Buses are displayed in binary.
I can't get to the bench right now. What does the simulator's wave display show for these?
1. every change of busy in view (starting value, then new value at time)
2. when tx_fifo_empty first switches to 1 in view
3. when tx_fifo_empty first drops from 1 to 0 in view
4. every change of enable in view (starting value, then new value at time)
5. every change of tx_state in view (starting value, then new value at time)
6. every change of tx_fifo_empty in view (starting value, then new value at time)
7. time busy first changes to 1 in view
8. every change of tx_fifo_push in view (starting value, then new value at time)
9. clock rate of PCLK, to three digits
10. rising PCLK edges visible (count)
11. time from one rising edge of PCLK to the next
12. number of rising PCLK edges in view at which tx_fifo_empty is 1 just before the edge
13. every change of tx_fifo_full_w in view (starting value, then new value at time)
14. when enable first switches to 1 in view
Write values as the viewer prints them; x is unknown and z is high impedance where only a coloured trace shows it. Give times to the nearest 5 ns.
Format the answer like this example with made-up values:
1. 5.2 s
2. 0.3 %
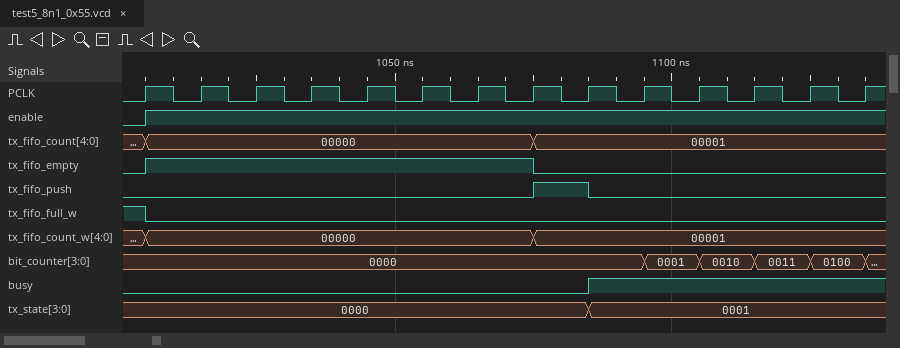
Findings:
1. 0, 1 at 1085 ns
2. 1005 ns
3. 1075 ns
4. 0, 1 at 1005 ns
5. 0000, 0001 at 1085 ns
6. 0, 1 at 1005 ns, 0 at 1075 ns
7. 1085 ns
8. 0, 1 at 1075 ns, 0 at 1085 ns
9. 100 MHz
10. 14
11. 10 ns
12. 7
13. 1, 0 at 1005 ns
14. 1005 ns
